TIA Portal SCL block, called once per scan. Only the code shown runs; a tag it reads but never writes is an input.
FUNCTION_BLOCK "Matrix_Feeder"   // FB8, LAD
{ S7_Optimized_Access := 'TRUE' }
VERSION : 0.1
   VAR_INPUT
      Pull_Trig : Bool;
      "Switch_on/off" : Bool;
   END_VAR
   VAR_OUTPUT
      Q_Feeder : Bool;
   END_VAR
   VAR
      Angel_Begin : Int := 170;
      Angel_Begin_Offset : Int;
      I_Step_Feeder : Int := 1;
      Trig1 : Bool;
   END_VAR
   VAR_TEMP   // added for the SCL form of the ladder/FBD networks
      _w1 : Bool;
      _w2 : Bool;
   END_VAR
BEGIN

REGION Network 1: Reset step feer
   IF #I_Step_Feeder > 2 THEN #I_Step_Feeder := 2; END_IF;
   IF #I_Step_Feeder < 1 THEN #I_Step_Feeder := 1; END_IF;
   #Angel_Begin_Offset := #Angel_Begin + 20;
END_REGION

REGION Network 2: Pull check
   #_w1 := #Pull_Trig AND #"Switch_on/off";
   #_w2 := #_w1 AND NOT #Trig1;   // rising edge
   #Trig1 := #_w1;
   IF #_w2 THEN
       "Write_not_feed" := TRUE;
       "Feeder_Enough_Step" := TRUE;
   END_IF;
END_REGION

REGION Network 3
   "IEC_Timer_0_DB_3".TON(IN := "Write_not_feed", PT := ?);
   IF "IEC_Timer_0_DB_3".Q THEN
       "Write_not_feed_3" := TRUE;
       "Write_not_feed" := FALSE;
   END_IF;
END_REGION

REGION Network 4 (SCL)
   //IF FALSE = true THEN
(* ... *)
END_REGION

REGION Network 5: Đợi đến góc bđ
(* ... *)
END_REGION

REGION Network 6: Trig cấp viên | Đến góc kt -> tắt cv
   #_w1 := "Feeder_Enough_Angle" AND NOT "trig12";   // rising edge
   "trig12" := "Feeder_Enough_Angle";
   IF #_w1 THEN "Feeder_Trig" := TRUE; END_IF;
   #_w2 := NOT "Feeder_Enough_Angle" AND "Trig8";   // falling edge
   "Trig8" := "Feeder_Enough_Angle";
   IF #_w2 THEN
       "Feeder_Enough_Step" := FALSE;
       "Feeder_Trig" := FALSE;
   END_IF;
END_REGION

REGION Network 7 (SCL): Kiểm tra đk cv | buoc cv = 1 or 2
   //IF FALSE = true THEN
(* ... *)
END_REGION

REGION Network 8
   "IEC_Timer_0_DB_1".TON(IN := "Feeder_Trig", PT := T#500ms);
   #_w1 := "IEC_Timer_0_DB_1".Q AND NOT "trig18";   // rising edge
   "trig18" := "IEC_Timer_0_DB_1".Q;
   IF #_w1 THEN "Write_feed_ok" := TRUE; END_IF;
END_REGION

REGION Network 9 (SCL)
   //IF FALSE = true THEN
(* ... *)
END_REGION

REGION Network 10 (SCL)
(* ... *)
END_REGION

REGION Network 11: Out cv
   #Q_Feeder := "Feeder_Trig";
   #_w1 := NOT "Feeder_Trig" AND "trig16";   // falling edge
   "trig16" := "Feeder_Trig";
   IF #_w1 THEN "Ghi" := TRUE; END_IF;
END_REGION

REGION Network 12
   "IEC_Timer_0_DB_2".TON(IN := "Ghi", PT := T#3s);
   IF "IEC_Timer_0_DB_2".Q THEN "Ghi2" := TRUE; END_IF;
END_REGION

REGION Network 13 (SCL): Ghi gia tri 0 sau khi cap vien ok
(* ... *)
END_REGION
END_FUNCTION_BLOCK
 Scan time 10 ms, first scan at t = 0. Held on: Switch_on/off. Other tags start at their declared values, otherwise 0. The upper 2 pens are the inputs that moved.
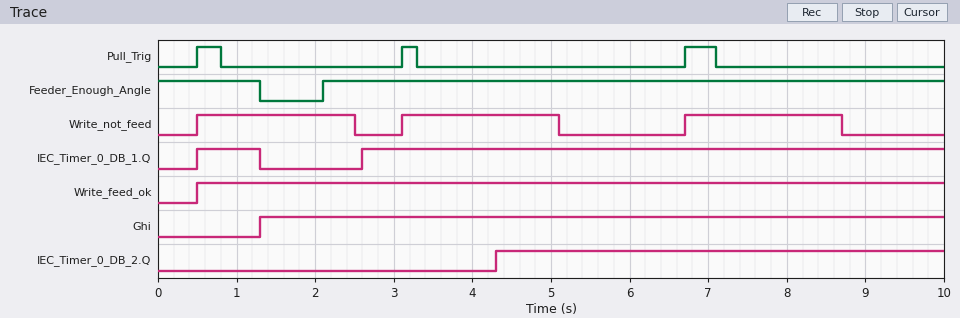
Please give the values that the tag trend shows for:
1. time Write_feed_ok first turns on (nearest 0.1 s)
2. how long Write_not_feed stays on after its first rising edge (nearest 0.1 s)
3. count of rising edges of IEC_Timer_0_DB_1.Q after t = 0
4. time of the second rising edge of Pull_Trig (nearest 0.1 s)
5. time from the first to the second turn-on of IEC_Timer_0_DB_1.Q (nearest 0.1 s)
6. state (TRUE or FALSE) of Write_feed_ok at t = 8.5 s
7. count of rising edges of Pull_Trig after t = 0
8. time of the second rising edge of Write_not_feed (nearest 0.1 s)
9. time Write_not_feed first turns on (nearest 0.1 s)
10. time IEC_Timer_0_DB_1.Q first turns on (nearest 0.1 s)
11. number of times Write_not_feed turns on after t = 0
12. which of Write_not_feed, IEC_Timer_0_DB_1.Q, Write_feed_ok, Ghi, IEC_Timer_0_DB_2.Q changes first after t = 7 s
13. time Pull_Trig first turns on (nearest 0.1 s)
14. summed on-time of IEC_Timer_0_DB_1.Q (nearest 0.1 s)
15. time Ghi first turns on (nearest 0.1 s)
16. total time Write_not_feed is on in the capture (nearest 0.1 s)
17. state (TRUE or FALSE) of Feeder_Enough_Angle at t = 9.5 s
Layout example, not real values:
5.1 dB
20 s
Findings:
0.5 s
2.0 s
2
3.1 s
2.1 s
TRUE
3
3.1 s
0.5 s
0.5 s
3
Write_not_feed
0.5 s
8.2 s
1.3 s
6.0 s
TRUE
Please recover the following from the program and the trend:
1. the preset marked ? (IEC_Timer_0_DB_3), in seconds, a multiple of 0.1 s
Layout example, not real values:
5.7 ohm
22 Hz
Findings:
2.0 s
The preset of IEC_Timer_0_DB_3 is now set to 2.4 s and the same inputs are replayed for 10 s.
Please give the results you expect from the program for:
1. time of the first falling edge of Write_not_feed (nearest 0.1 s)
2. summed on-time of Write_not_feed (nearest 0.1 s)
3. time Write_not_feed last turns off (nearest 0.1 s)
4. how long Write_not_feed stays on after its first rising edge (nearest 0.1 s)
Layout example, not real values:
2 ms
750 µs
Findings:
2.9 s
7.2 s
9.1 s
2.4 s
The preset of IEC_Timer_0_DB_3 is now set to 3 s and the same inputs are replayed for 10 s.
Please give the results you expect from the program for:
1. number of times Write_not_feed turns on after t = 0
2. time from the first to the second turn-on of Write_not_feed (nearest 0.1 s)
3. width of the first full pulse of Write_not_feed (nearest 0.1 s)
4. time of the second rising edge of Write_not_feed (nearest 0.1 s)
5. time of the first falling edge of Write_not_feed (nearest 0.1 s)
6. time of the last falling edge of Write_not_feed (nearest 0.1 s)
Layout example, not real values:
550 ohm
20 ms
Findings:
2
6.2 s
3.0 s
6.7 s
3.5 s
9.7 s
